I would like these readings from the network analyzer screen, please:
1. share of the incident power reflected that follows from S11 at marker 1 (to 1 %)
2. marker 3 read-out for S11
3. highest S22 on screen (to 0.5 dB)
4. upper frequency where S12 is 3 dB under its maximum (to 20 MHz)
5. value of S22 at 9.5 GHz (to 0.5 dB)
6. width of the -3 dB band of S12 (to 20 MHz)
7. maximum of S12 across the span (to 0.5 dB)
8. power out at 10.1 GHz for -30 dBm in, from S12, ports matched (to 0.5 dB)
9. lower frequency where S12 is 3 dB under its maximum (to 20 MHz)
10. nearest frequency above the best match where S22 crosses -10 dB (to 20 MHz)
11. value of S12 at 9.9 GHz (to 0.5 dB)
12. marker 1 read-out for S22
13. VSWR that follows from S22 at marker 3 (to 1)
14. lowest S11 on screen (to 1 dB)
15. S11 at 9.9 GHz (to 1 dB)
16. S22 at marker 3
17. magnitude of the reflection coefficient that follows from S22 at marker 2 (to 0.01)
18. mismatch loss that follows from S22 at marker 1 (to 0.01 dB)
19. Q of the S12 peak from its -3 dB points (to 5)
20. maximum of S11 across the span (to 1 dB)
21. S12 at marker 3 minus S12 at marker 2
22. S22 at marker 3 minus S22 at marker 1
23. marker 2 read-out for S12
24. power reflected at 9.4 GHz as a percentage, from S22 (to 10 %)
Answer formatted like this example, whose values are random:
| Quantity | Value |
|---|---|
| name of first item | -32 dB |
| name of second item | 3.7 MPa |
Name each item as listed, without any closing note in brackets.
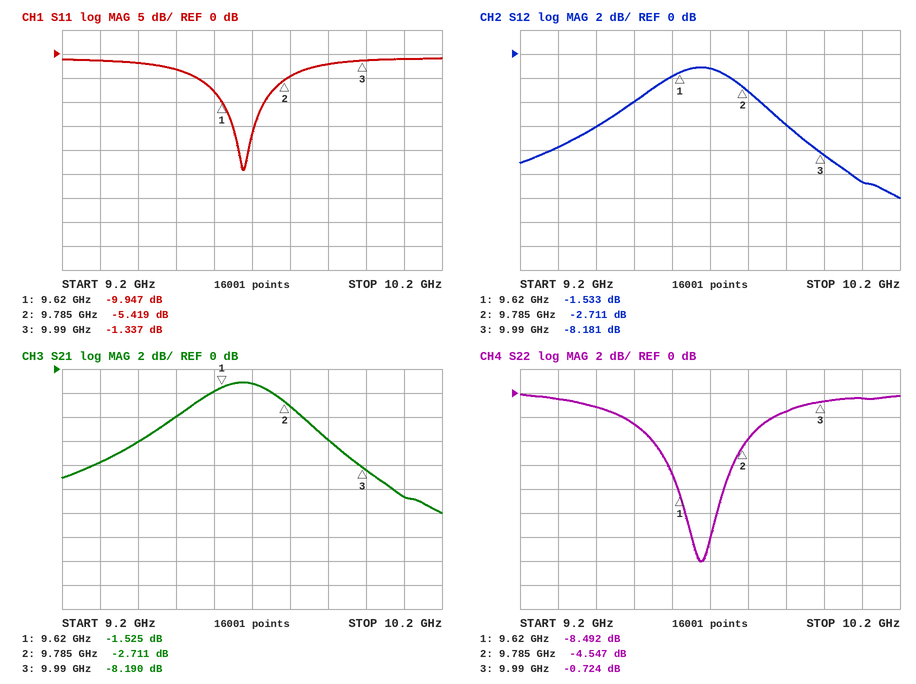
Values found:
| Quantity | Value |
|---|---|
| share of the incident power reflected that follows from S11 at marker 1 | 10 % |
| marker 3 read-out for S11 | -1.337 dB |
| highest S22 on screen | 0.0 dB |
| upper frequency where S12 is 3 dB under its maximum | 9.84 GHz |
| value of S22 at 9.5 GHz | -2.5 dB |
| width of the -3 dB band of S12 | 340 MHz |
| maximum of S12 across the span | -1.0 dB |
| power out at 10.1 GHz for -30 dBm in, from S12, ports matched | -40.5 dBm |
| lower frequency where S12 is 3 dB under its maximum | 9.50 GHz |
| nearest frequency above the best match where S22 crosses -10 dB | 9.72 GHz |
| value of S12 at 9.9 GHz | -6.0 dB |
| marker 1 read-out for S22 | -8.492 dB |
| VSWR that follows from S22 at marker 3 | 24 |
| lowest S11 on screen | -24 dB |
| S11 at 9.9 GHz | -2 dB |
| S22 at marker 3 | -0.724 dB |
| magnitude of the reflection coefficient that follows from S22 at marker 2 | 0.59 |
| mismatch loss that follows from S22 at marker 1 | 0.66 dB |
| Q of the S12 peak from its -3 dB points | 30 |
| maximum of S11 across the span | -1 dB |
| S12 at marker 3 minus S12 at marker 2 | -5.470 dB |
| S22 at marker 3 minus S22 at marker 1 | 7.768 dB |
| marker 2 read-out for S12 | -2.711 dB |
| power reflected at 9.4 GHz as a percentage, from S22 | 80 % |
